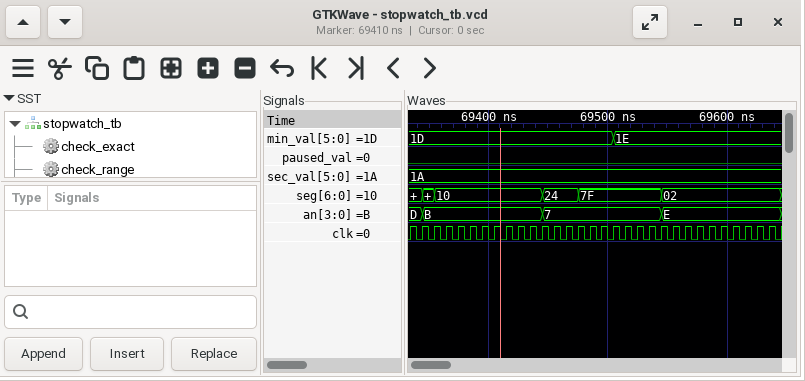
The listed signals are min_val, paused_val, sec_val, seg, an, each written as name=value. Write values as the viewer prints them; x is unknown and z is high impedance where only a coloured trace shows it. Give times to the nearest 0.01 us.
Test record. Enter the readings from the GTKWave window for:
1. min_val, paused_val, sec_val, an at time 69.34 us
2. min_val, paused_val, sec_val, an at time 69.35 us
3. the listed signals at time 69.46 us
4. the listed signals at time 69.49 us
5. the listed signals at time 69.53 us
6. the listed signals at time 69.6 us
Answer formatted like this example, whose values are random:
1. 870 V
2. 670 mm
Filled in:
1. min_val=1D, paused_val=0, sec_val=1A, an=D
2. min_val=1D, paused_val=0, sec_val=1A, an=B
3. min_val=1D, paused_val=0, sec_val=1A, seg=24, an=7
4. min_val=1D, paused_val=0, sec_val=1A, seg=7F, an=7
5. min_val=1E, paused_val=0, sec_val=1A, seg=7F, an=7
6. min_val=1E, paused_val=0, sec_val=1A, seg=02, an=E
